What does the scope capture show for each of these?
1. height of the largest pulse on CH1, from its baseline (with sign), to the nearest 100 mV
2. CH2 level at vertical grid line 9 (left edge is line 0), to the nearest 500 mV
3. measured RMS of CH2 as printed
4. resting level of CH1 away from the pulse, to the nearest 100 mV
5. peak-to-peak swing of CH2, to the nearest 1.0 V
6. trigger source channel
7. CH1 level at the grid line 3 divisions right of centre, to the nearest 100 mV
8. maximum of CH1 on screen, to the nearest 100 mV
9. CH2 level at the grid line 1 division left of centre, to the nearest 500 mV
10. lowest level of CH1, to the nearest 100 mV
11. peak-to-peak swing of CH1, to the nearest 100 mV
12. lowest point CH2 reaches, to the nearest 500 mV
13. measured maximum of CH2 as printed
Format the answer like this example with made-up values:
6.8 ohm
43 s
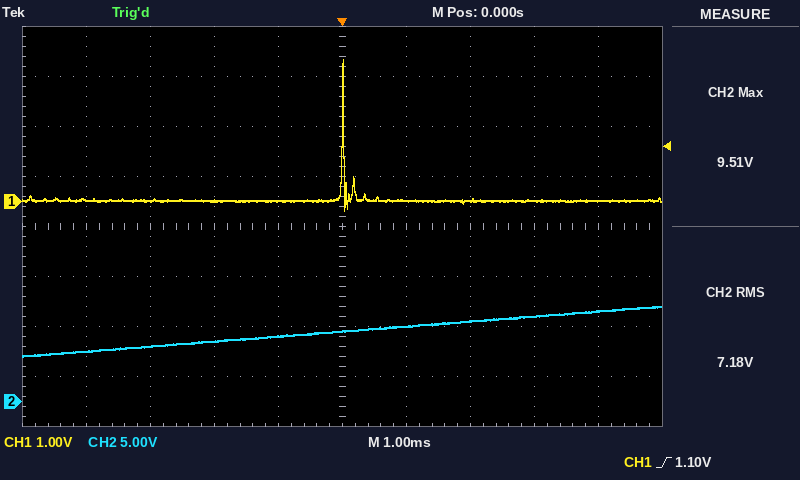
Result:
+2.8 V
9.0 V
7.18 V
0.0 V
5.0 V
CH1
0.0 V
2.8 V
6.5 V
-200 mV
3.0 V
4.5 V
9.51 V
